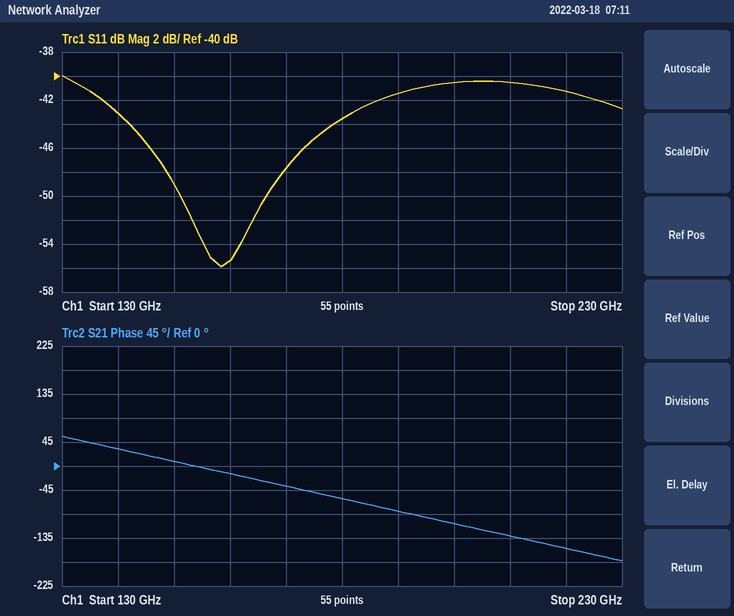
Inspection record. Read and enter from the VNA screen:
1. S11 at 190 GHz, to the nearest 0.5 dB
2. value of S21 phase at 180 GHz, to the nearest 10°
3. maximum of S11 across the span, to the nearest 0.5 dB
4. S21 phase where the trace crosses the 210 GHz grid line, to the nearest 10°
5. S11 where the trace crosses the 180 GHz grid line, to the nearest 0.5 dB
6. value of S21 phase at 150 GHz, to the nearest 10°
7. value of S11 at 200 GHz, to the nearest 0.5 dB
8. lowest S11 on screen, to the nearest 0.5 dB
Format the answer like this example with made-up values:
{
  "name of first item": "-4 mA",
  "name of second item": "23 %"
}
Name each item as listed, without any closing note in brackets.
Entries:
{
  "S11 at 190 GHz, to the nearest 0.5 dB": "-41.5 dB",
  "value of S21 phase at 180 GHz, to the nearest 10°": "-60°",
  "maximum of S11 across the span, to the nearest 0.5 dB": "-40.0 dB",
  "S21 phase where the trace crosses the 210 GHz grid line, to the nearest 10°": "-130°",
  "S11 where the trace crosses the 180 GHz grid line, to the nearest 0.5 dB": "-43.5 dB",
  "value of S21 phase at 150 GHz, to the nearest 10°": "10°",
  "value of S11 at 200 GHz, to the nearest 0.5 dB": "-40.5 dB",
  "lowest S11 on screen, to the nearest 0.5 dB": "-56.0 dB"
}
